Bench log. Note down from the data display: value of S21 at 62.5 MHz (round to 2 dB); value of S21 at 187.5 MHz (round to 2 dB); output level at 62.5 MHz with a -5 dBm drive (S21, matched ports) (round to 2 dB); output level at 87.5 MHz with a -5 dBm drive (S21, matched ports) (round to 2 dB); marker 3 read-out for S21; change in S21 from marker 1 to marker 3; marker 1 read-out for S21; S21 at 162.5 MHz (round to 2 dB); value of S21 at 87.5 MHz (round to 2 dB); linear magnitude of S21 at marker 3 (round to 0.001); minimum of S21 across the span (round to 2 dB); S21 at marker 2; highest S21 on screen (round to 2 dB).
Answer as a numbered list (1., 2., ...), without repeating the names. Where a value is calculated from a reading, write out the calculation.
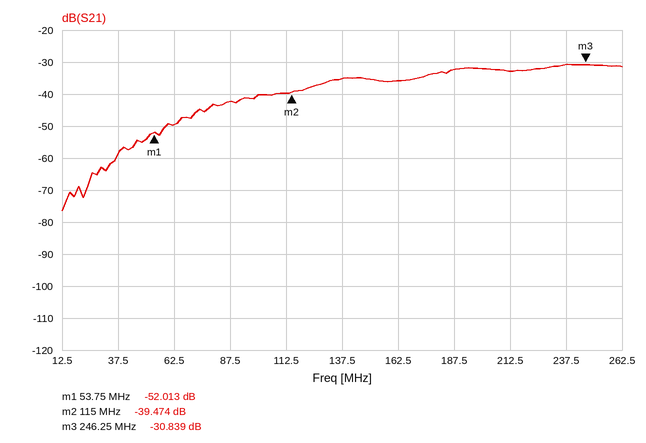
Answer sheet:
1. -50 dB
2. -32 dB
3. -5 dBm + (-50 dB) = -54 dBm
4. -5 dBm + (-42 dB) = -48 dBm
5. -30.839 dB
6. -30.839 − (-52.013) = 21.174 dB
7. -52.013 dB
8. -36 dB
9. -42 dB
10. 10^(-30.839/20) ≈ 0.029
11. -76 dB
12. -39.474 dB
13. -30 dB
